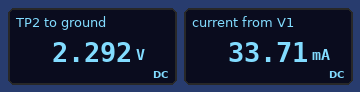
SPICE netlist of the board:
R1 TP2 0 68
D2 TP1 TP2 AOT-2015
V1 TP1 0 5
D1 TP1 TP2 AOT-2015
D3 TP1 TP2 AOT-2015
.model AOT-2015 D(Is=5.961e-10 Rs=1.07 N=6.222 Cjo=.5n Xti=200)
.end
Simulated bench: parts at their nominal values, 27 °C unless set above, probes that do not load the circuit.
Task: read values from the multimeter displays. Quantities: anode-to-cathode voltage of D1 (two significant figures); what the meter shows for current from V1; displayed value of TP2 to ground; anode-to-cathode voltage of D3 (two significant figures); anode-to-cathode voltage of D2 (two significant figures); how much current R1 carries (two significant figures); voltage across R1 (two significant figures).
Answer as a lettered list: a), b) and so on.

a) 2.7 V
b) 33.71 mA
c) 2.292 V
d) 2.7 V
e) 2.7 V
f) 34 mA
g) 2.3 V
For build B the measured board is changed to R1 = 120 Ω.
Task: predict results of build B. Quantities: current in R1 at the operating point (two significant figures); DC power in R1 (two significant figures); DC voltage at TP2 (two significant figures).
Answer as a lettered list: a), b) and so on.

a) 20 mA
b) 47 mW
c) 2.4 V
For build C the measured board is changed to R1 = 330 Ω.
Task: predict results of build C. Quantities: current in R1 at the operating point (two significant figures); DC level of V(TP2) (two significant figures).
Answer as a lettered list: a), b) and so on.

a) 7.7 mA
b) 2.5 V
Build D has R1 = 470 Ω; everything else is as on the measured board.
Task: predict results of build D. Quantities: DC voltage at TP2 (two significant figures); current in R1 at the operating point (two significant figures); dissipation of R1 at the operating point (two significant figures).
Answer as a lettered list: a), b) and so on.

a) 2.6 V
b) 5.5 mA
c) 14 mW
